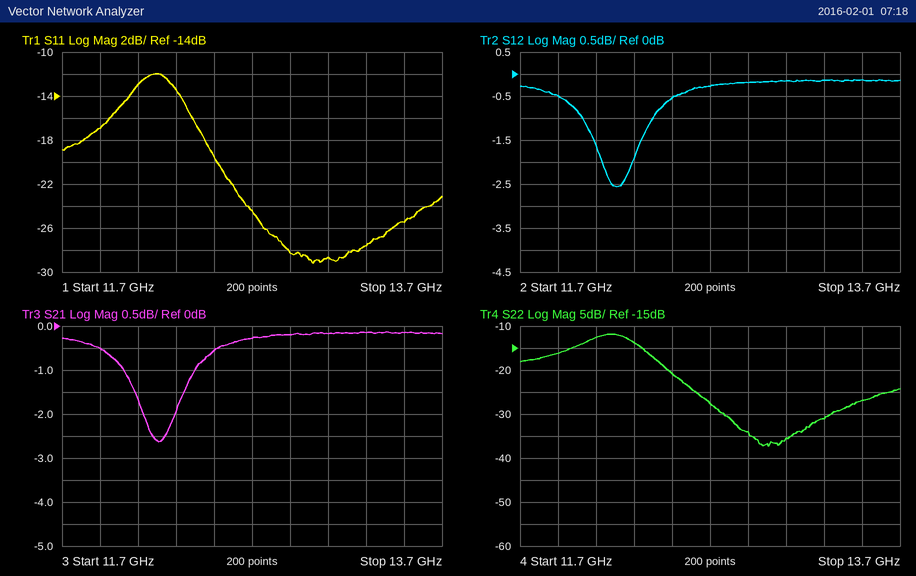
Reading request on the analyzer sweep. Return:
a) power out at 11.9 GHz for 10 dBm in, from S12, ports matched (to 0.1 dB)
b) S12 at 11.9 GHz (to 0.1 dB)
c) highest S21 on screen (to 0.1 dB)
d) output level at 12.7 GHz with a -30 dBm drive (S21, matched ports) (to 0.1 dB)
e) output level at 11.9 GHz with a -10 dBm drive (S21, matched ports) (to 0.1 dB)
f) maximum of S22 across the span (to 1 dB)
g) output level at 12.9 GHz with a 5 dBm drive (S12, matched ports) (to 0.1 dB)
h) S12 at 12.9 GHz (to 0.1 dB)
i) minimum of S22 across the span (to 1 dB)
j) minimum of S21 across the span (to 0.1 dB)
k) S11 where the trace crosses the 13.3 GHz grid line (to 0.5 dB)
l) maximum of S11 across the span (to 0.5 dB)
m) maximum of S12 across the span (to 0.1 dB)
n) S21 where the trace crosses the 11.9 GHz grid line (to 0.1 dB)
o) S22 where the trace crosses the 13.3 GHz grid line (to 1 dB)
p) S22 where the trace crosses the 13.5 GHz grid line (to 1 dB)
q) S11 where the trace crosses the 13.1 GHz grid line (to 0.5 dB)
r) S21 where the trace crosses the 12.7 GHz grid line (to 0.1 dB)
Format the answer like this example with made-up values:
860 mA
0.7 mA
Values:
9.5 dBm
-0.5 dB
-0.1 dB
-30.3 dBm
-10.5 dBm
-12 dB
4.8 dBm
-0.2 dB
-37 dB
-2.6 dB
-27.5 dB
-12.0 dB
-0.1 dB
-0.5 dB
-31 dB
-27 dB
-28.5 dB
-0.3 dB
